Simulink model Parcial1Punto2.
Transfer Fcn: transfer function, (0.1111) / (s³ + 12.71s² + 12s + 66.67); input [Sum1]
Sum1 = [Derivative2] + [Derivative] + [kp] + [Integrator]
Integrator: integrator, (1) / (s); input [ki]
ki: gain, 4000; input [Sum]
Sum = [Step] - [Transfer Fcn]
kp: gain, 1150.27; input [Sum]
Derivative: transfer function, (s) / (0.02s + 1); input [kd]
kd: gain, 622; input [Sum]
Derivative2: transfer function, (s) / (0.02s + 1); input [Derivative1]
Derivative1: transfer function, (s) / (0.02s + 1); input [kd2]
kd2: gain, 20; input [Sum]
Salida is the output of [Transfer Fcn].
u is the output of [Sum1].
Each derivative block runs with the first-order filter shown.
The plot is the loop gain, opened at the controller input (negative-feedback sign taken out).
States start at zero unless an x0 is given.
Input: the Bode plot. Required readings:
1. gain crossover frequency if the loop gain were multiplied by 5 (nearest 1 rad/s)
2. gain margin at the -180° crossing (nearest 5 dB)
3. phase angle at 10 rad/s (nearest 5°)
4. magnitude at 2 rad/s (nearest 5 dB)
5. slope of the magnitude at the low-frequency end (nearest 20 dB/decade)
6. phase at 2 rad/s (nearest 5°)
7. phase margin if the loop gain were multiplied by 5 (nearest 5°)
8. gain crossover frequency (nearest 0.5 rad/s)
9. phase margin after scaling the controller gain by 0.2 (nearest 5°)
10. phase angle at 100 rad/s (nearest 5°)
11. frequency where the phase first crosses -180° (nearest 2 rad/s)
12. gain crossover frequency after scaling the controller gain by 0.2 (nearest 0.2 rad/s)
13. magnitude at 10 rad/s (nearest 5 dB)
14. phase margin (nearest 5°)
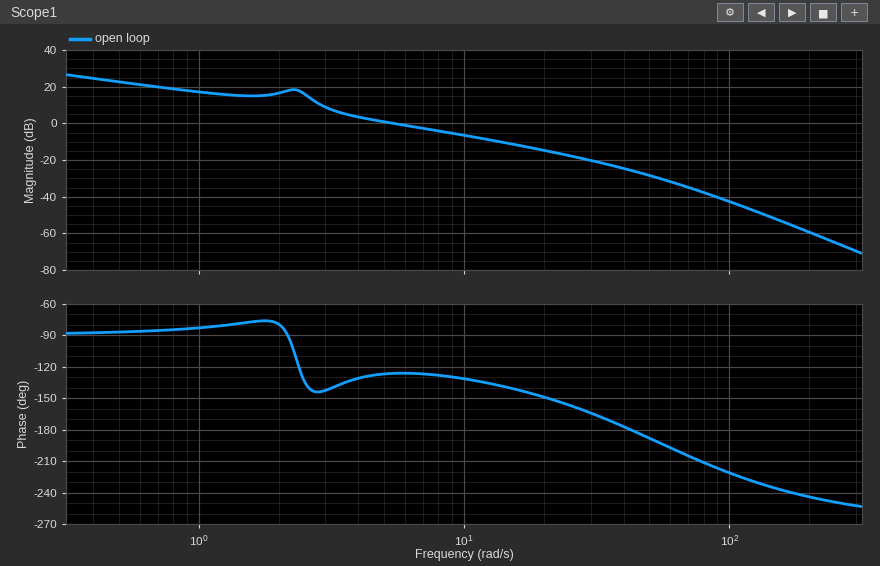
19 rad/s
25 dB
-130°
15 dB
-20 dB/decade
-80°
35°
5.5 rad/s
40°
-220°
42 rad/s
2.6 rad/s
-5 dB
55°
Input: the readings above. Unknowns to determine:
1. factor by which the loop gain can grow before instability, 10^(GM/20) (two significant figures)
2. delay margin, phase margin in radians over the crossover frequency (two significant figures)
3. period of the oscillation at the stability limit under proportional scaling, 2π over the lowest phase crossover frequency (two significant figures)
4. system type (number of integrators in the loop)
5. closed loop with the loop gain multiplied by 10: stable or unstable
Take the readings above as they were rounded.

18
0.17 s
0.15 s
1
stable
